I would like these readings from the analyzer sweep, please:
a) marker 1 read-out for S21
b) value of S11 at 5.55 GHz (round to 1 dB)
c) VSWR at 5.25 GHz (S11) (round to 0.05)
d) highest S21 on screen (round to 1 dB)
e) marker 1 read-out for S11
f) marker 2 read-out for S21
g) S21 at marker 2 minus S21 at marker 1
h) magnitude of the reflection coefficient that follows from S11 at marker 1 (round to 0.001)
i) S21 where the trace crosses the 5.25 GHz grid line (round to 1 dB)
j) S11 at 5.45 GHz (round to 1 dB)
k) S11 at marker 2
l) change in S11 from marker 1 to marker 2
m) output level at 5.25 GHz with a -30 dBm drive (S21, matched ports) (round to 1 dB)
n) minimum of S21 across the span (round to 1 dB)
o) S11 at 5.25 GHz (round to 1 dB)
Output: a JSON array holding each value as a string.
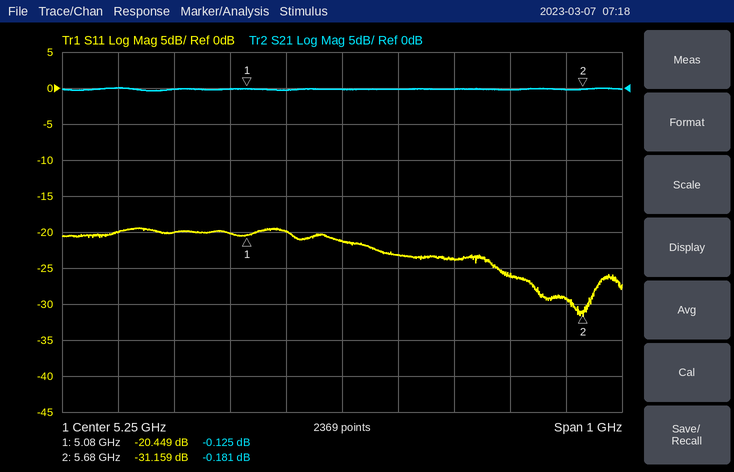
["-0.125 dB", "-26 dB", "1.20", "0 dB", "-20.449 dB", "-0.181 dB", "-0.056 dB", "0.095", "0 dB", "-24 dB", "-31.159 dB", "-10.710 dB", "-30 dBm", "0 dB", "-21 dB"]
